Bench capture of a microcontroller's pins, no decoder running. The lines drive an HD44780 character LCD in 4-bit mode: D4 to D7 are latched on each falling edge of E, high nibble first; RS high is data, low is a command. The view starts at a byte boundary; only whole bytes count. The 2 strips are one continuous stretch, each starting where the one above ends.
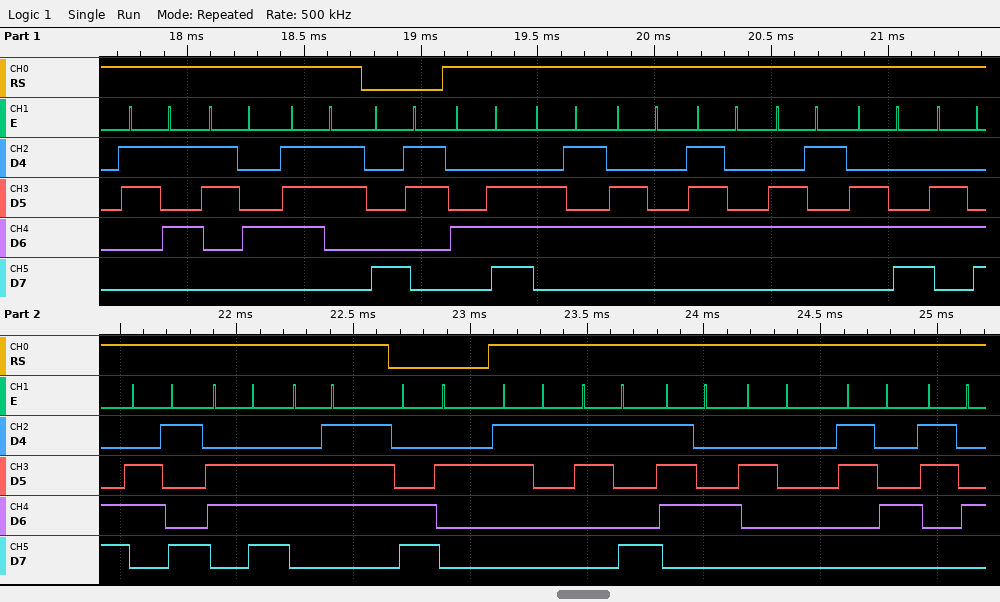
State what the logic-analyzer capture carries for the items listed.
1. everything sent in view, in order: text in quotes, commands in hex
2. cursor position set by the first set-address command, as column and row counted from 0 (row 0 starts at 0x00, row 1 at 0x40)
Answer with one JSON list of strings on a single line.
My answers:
["\"54s\" 0x83 \"Nedtelling\" 0xC2 \"19t 44\"", "column 3, row 0"]
